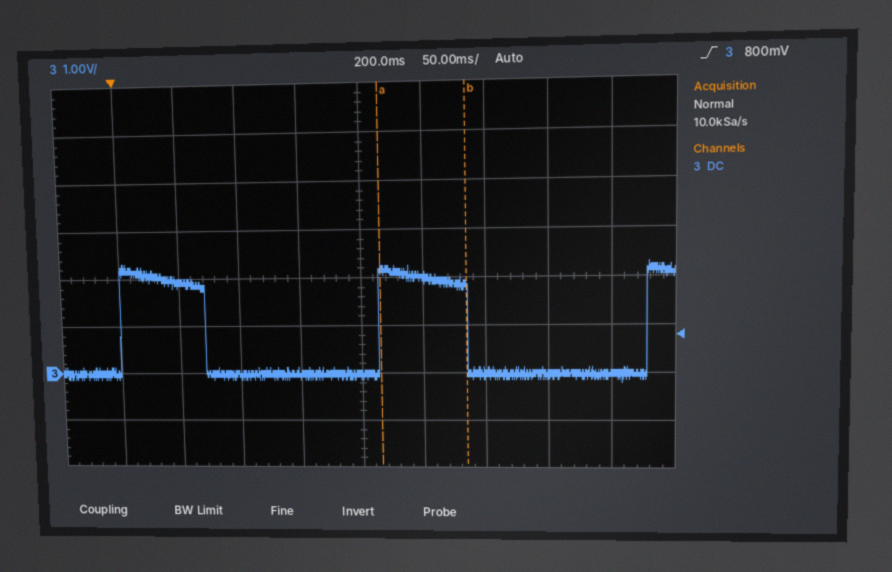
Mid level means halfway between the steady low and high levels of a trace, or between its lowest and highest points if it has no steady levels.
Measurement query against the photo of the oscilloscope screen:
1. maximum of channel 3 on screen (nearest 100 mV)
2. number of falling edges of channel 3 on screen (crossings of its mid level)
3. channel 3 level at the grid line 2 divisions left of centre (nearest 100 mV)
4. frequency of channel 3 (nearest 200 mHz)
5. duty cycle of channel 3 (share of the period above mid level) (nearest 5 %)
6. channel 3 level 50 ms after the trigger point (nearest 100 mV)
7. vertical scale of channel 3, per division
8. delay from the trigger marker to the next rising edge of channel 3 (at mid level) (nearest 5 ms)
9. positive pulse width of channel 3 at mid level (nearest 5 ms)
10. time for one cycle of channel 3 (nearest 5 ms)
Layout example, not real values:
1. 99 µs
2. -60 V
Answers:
1. 2.3 V
2. 2
3. 0.0 V
4. 4.6 Hz
5. 35 %
6. 1.9 V
7. 1 V
8. 215 ms
9. 70 ms
10. 215 ms
